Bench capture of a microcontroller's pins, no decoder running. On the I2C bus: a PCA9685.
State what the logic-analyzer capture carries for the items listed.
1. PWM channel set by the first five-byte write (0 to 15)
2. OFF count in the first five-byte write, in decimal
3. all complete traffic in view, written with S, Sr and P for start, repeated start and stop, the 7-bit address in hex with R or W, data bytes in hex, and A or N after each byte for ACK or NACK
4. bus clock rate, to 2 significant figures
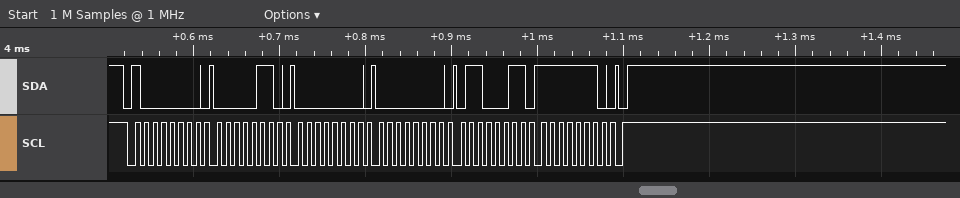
0
65123
S 40W A 06 A 00 A 00 A 63 A FE A P
100 kHz
